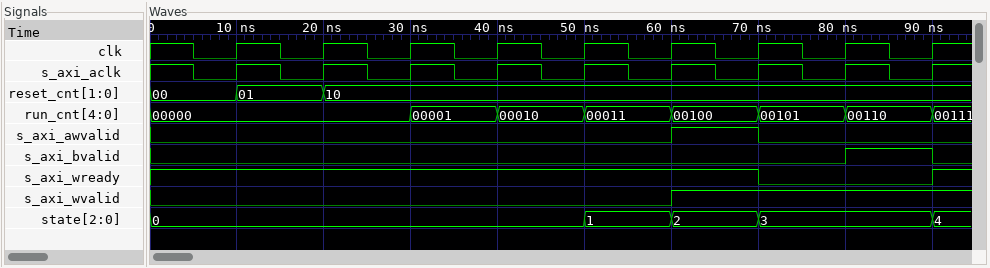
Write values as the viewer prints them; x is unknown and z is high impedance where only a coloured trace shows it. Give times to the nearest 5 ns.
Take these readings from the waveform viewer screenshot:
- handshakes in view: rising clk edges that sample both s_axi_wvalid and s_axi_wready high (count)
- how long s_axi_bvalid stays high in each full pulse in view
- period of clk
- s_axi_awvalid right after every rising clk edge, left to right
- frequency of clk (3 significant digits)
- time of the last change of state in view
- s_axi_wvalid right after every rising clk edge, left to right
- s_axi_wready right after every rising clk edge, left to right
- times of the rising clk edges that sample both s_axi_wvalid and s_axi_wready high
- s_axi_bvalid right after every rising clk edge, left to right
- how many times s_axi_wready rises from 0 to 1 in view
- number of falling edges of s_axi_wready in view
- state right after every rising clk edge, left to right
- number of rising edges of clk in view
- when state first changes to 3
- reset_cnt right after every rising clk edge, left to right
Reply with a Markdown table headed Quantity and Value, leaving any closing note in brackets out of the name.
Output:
| Quantity | Value |
|---|---|
| handshakes in view: rising clk edges that sample both s_axi_wvalid and s_axi_wready high | 1 |
| how long s_axi_bvalid stays high in each full pulse in view | 10 ns |
| period of clk | 10 ns |
| s_axi_awvalid right after every rising clk edge, left to right | 0 0 0 0 0 1 0 0 0 |
| frequency of clk | 100 MHz |
| time of the last change of state in view | 90 ns |
| s_axi_wvalid right after every rising clk edge, left to right | 0 0 0 0 0 1 1 1 1 |
| s_axi_wready right after every rising clk edge, left to right | 1 1 1 1 1 1 0 0 1 |
| times of the rising clk edges that sample both s_axi_wvalid and s_axi_wready high | 70 ns |
| s_axi_bvalid right after every rising clk edge, left to right | 0 0 0 0 0 0 0 1 0 |
| how many times s_axi_wready rises from 0 to 1 in view | 1 |
| number of falling edges of s_axi_wready in view | 1 |
| state right after every rising clk edge, left to right | 0, 0, 0, 0, 1, 2, 3, 3, 4 |
| number of rising edges of clk in view | 9 |
| when state first changes to 3 | 70 ns |
| reset_cnt right after every rising clk edge, left to right | 01, 10, 10, 10, 10, 10, 10, 10, 10 |
